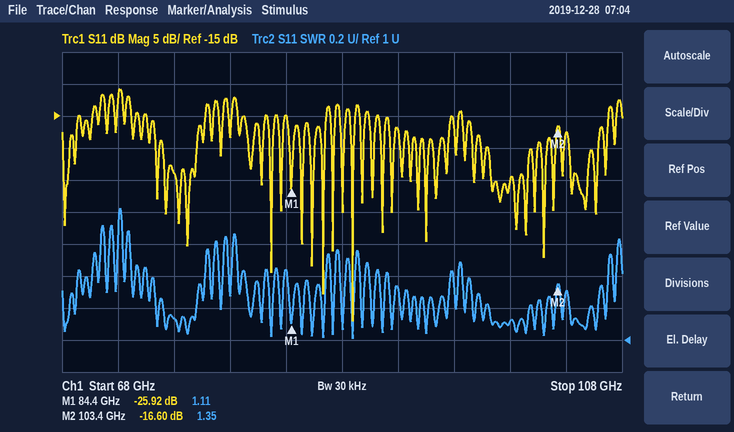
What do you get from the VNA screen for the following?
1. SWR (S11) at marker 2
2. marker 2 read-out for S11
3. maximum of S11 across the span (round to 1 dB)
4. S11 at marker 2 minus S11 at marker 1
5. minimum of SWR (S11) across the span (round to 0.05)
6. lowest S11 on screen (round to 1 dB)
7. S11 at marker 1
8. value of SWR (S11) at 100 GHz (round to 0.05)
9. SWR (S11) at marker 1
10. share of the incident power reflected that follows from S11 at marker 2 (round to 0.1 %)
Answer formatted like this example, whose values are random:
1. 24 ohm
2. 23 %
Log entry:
1. 1.35
2. -16.60 dB
3. -11 dB
4. 9.32 dB
5. 1.00
6. -47 dB
7. -25.92 dB
8. 1.10
9. 1.11
10. 2.2 %
